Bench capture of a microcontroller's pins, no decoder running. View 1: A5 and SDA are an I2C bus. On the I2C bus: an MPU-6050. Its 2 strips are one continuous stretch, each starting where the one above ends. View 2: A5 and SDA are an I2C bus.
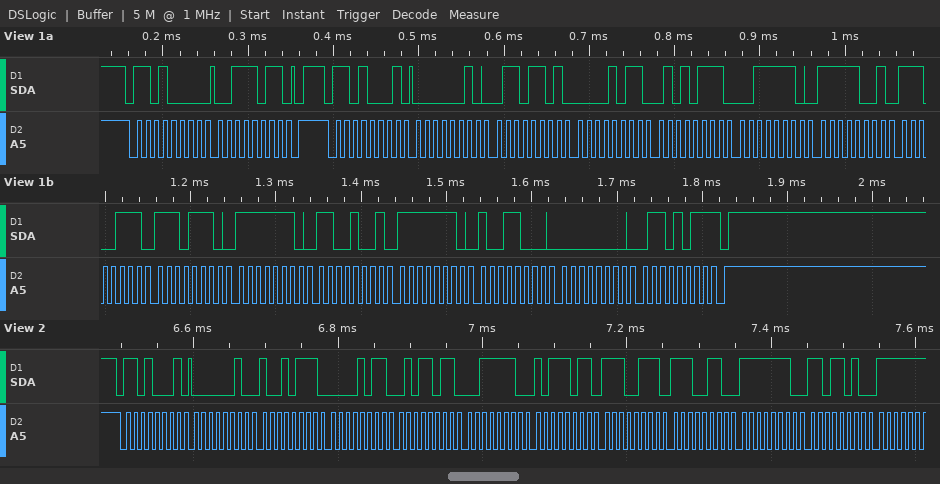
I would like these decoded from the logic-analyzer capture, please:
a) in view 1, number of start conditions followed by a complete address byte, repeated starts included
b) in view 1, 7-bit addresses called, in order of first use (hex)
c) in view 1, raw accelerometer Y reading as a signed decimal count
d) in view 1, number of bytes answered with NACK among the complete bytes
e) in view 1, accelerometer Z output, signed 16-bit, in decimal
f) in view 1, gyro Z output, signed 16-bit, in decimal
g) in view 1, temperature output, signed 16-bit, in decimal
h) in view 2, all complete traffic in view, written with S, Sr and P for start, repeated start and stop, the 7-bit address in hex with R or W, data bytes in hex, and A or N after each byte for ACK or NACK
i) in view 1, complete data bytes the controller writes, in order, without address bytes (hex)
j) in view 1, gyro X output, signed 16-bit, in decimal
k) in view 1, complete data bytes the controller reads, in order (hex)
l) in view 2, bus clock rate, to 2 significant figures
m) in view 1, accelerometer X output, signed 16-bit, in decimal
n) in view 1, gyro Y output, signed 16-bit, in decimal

2
0x68
2903
1
16121
107
-6162
S 68R A 02 A 97 A 0B A 5B A 3E A BB A E7 A E6 A FE A DA A
3B
-311
02 6D 0B 57 3E F9 E7 EE FE C9 FE 98 00 6B
100 kHz
621
-360
